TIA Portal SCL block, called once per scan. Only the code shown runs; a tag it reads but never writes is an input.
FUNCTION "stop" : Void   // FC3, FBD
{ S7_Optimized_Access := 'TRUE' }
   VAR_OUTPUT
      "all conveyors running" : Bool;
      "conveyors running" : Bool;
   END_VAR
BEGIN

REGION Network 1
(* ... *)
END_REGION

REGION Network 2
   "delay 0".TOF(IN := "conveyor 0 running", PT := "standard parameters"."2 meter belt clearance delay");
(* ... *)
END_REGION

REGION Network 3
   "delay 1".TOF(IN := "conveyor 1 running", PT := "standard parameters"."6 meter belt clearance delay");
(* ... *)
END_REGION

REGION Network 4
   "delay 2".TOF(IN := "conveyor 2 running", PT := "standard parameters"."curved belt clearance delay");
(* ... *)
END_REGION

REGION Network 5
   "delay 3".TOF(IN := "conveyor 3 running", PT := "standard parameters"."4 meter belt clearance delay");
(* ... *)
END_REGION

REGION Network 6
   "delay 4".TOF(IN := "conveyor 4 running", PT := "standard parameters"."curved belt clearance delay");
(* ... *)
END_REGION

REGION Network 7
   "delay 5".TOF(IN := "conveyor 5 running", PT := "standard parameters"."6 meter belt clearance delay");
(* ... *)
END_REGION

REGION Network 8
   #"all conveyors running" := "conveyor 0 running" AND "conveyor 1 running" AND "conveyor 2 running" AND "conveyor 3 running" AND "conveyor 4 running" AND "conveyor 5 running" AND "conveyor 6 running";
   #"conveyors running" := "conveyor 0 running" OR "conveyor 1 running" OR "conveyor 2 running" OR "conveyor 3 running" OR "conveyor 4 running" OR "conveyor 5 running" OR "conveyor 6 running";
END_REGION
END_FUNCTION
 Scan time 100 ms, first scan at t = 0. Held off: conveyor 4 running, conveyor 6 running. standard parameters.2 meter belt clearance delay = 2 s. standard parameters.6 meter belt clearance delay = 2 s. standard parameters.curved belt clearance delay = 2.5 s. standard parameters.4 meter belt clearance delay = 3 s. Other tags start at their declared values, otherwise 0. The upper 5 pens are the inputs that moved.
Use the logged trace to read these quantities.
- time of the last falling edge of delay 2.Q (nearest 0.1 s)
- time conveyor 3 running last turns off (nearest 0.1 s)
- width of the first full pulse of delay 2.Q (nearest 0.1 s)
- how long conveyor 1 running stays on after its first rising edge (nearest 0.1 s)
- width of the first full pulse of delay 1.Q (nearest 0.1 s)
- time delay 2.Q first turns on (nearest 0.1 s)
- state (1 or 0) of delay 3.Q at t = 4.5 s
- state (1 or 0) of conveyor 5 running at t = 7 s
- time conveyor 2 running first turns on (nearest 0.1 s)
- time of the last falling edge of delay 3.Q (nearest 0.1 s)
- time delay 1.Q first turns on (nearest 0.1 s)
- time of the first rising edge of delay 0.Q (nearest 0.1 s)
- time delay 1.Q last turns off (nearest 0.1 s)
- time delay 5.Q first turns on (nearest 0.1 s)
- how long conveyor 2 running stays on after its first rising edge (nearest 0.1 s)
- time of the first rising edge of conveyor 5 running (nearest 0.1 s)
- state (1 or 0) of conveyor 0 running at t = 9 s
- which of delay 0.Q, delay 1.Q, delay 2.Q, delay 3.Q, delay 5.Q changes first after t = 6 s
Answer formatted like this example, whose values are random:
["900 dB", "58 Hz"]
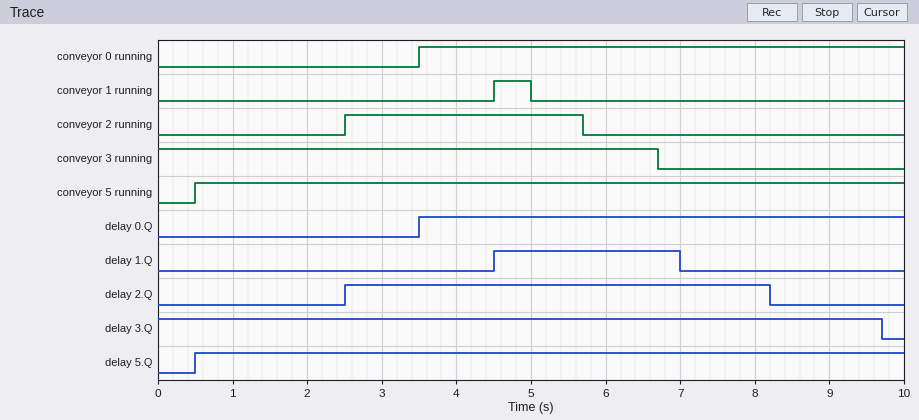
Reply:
["8.2 s", "6.7 s", "5.7 s", "0.5 s", "2.5 s", "2.5 s", "1", "1", "2.5 s", "9.7 s", "4.5 s", "3.5 s", "7.0 s", "0.5 s", "3.2 s", "0.5 s", "1", "delay 1.Q"]
